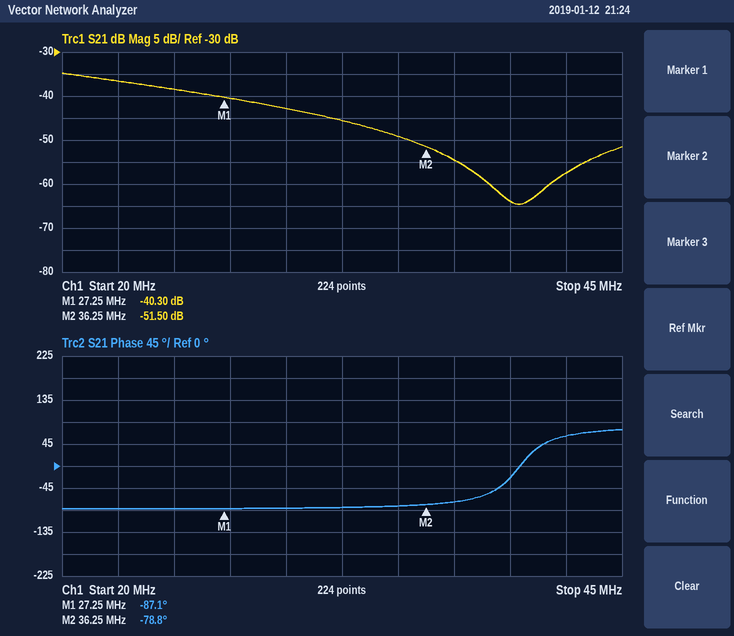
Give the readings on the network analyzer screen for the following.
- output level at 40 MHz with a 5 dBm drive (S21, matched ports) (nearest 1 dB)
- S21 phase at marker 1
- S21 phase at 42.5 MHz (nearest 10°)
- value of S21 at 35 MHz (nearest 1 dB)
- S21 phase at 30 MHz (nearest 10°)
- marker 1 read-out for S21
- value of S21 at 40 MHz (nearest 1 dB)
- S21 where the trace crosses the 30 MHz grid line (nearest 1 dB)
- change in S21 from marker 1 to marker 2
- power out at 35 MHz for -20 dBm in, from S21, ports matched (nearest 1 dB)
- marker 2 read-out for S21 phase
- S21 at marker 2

-59 dBm
-87.1°
60°
-49 dB
-90°
-40.30 dB
-64 dB
-43 dB
-11.20 dB
-69 dBm
-78.8°
-51.50 dB
